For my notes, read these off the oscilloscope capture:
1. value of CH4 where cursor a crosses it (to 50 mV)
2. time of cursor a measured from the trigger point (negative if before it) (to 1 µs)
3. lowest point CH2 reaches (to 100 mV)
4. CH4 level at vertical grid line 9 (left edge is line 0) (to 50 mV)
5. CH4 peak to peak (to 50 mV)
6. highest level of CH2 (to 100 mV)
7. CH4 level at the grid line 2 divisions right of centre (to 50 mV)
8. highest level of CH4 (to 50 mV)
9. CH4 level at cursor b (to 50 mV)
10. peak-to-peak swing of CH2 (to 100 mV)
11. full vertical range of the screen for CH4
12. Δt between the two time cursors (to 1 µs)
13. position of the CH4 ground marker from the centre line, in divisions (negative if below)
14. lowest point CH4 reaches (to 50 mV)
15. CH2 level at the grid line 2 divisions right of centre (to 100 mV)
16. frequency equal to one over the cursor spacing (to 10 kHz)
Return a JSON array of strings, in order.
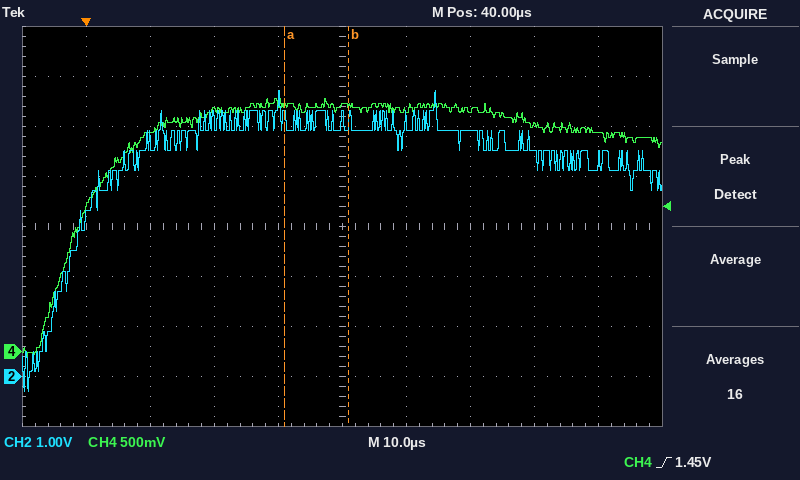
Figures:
["2.45 V", "+31 µs", "-300 mV", "2.20 V", "2.60 V", "5.7 V", "2.40 V", "2.55 V", "2.45 V", "6.0 V", "4 V", "10 µs", "-2.5 div", "-50 mV", "4.9 V", "100 kHz"]
